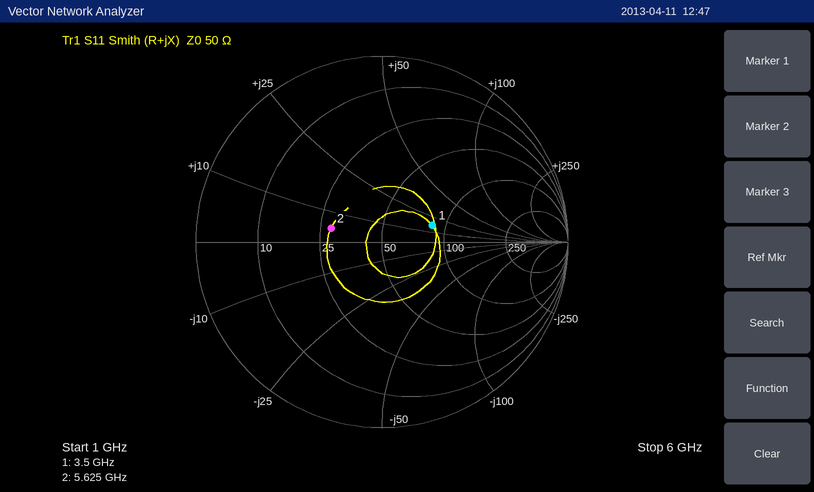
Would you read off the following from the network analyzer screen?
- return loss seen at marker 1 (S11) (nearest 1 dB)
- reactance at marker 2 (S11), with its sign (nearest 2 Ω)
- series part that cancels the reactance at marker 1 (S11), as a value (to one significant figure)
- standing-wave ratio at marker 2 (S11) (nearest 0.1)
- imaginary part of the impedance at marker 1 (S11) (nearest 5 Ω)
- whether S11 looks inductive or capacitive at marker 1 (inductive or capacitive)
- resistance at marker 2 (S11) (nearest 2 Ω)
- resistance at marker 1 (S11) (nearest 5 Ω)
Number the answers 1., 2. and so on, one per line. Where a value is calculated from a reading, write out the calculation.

1. 11 dB
2. +4 Ω
3. C = 1/(2π × 3.5 GHz × 15 Ω) ≈ 3 pF
4. 1.8
5. +15 Ω
6. inductive
7. 28 Ω
8. 85 Ω
